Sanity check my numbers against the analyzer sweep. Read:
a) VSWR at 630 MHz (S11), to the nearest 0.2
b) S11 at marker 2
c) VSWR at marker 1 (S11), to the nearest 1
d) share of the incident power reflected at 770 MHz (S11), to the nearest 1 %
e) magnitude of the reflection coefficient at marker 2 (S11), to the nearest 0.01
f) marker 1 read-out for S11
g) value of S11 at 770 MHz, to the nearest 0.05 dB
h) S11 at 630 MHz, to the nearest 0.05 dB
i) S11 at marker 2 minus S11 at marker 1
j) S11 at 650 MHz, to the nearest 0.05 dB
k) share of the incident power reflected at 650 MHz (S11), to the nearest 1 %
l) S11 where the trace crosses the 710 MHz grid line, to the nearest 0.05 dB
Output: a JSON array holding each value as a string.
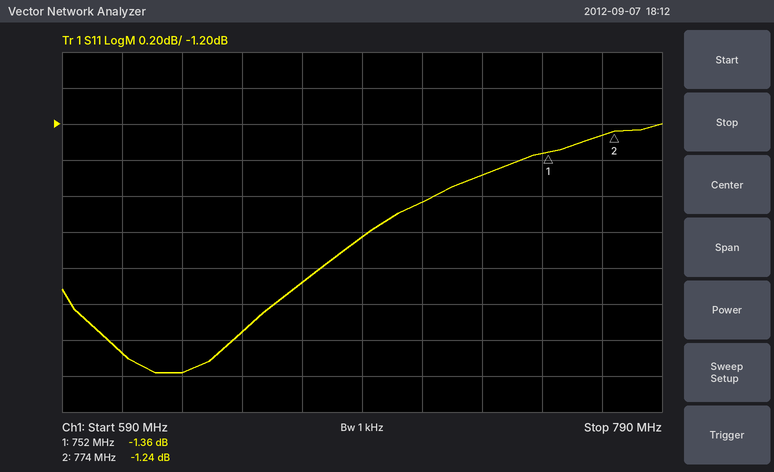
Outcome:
["6.8", "-1.24 dB", "13", "75 %", "0.87", "-1.36 dB", "-1.25 dB", "-2.60 dB", "0.12 dB", "-2.35 dB", "58 %", "-1.65 dB"]
